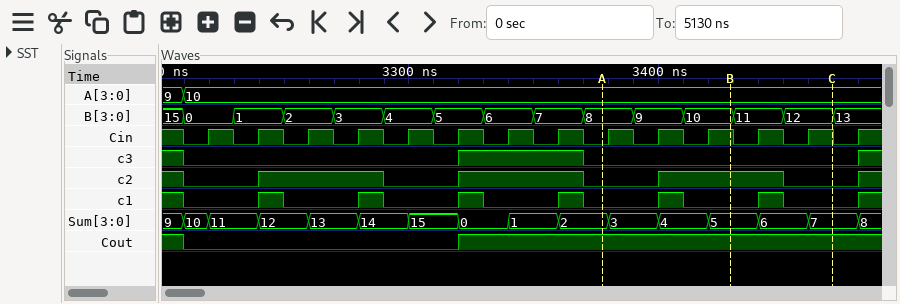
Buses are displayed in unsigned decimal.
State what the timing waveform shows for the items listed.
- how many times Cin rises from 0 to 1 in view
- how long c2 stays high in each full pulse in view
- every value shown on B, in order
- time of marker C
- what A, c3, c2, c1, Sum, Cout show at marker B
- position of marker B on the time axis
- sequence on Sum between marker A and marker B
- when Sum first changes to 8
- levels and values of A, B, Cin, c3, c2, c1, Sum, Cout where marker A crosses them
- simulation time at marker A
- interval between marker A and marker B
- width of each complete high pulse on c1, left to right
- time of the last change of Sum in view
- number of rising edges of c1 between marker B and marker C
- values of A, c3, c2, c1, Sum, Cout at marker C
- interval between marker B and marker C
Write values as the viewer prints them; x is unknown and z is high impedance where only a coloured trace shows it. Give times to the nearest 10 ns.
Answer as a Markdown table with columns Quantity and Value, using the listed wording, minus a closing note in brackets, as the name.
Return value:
| Quantity | Value |
|---|---|
| how many times Cin rises from 0 to 1 in view | 14 |
| how long c2 stays high in each full pulse in view | 50 ns, 50 ns, 50 ns |
| every value shown on B, in order | 15, 0, 1, 2, 3, 4, 5, 6, 7, 8, 9, 10, 11, 12, 13 |
| time of marker C | 3470 ns |
| what A, c3, c2, c1, Sum, Cout show at marker B | A=10, c3=0, c2=1, c1=0, Sum=5, Cout=1 |
| position of marker B on the time axis | 3430 ns |
| sequence on Sum between marker A and marker B | 2, 3, 4, 5 |
| when Sum first changes to 8 | 3480 ns |
| levels and values of A, B, Cin, c3, c2, c1, Sum, Cout where marker A crosses them | A=10, B=8, Cin=0, c3=0, c2=0, c1=0, Sum=2, Cout=1 |
| simulation time at marker A | 3380 ns |
| interval between marker A and marker B | 50 ns |
| width of each complete high pulse on c1, left to right | 10 ns, 10 ns, 10 ns, 10 ns, 10 ns, 10 ns |
| time of the last change of Sum in view | 3480 ns |
| number of rising edges of c1 between marker B and marker C | 1 |
| values of A, c3, c2, c1, Sum, Cout at marker C | A=10, c3=0, c2=0, c1=0, Sum=7, Cout=1 |
| interval between marker B and marker C | 40 ns |
